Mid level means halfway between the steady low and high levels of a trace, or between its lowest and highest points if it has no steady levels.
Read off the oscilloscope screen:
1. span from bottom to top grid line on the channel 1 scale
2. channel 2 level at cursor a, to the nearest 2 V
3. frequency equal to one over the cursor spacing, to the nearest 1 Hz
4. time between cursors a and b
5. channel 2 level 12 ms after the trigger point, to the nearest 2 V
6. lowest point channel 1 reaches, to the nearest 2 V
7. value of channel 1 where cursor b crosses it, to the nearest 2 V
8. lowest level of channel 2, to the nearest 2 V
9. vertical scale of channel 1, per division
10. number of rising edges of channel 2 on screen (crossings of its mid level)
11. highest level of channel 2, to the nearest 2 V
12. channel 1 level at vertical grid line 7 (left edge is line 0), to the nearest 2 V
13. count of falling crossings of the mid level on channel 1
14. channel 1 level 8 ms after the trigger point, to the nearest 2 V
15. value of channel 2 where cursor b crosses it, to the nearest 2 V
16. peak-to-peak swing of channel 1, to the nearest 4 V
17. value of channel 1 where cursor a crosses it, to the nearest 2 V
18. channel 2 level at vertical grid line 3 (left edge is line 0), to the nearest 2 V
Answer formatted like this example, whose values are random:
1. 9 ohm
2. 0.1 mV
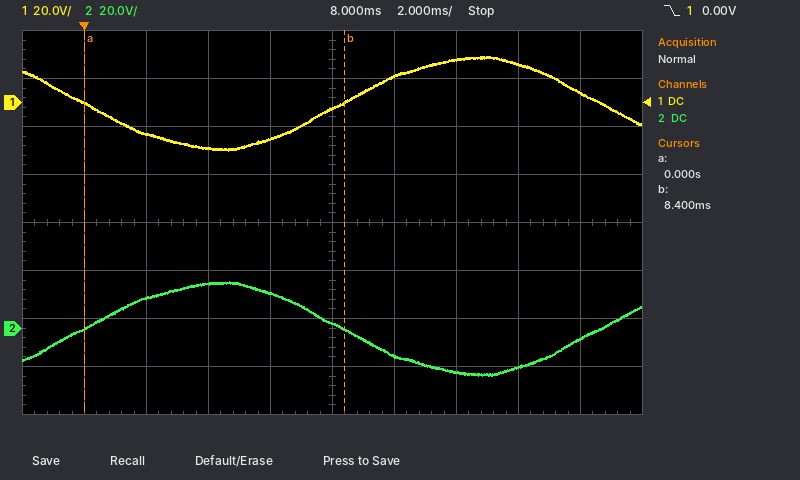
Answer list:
1. 160 V
2. 0 V
3. 119 Hz
4. 8.4 ms
5. -18 V
6. -20 V
7. 0 V
8. -20 V
9. 20 V
10. 2
11. 20 V
12. 18 V
13. 2
14. -2 V
15. 0 V
16. 40 V
17. 0 V
18. 18 V
